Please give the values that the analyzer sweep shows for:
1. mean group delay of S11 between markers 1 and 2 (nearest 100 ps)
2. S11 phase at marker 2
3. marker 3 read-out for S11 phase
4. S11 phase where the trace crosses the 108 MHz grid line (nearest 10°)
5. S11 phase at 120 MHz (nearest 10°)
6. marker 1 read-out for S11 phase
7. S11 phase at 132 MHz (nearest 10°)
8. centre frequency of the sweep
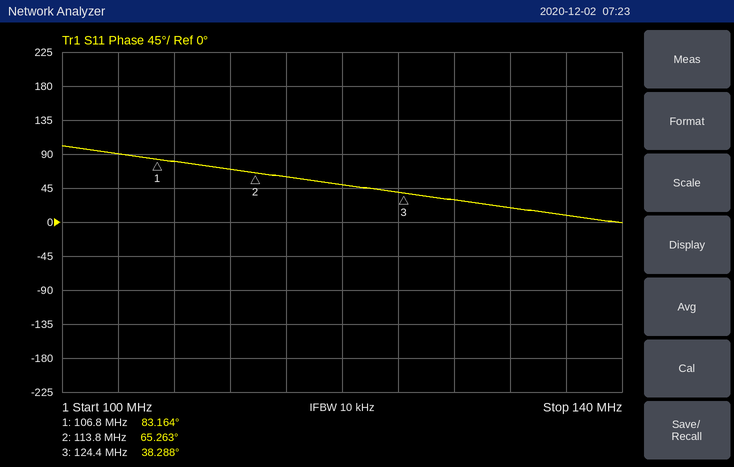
7.1 ns
65.263°
38.288°
80°
50°
83.164°
20°
120 MHz
